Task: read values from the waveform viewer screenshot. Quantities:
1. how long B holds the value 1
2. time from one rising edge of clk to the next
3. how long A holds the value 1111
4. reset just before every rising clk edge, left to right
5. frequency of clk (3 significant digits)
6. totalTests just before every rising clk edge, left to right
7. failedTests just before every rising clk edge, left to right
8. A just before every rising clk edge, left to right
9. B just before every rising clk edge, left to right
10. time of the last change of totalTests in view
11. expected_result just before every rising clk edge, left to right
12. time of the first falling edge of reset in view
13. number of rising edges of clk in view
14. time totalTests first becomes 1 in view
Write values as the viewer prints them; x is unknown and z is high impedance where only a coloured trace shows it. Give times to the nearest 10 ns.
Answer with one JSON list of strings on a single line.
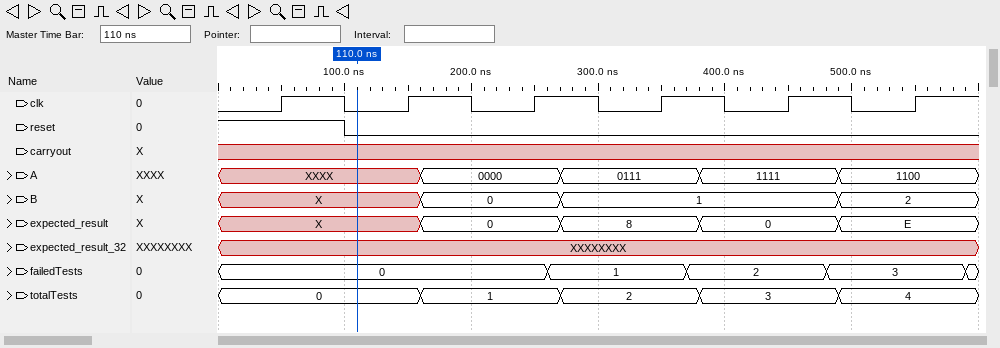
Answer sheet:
["220 ns", "100 ns", "110 ns", "1 0 0 0 0 0", "10.0 MHz", "0, 0, 1, 2, 3, 4", "0, 0, 0, 1, 2, 3", "XXXX, XXXX, 0000, 0111, 1111, 1100", "X, X, 0, 1, 1, 2", "490 ns", "X, X, 0, 8, 0, E", "100 ns", "6", "160 ns"]
